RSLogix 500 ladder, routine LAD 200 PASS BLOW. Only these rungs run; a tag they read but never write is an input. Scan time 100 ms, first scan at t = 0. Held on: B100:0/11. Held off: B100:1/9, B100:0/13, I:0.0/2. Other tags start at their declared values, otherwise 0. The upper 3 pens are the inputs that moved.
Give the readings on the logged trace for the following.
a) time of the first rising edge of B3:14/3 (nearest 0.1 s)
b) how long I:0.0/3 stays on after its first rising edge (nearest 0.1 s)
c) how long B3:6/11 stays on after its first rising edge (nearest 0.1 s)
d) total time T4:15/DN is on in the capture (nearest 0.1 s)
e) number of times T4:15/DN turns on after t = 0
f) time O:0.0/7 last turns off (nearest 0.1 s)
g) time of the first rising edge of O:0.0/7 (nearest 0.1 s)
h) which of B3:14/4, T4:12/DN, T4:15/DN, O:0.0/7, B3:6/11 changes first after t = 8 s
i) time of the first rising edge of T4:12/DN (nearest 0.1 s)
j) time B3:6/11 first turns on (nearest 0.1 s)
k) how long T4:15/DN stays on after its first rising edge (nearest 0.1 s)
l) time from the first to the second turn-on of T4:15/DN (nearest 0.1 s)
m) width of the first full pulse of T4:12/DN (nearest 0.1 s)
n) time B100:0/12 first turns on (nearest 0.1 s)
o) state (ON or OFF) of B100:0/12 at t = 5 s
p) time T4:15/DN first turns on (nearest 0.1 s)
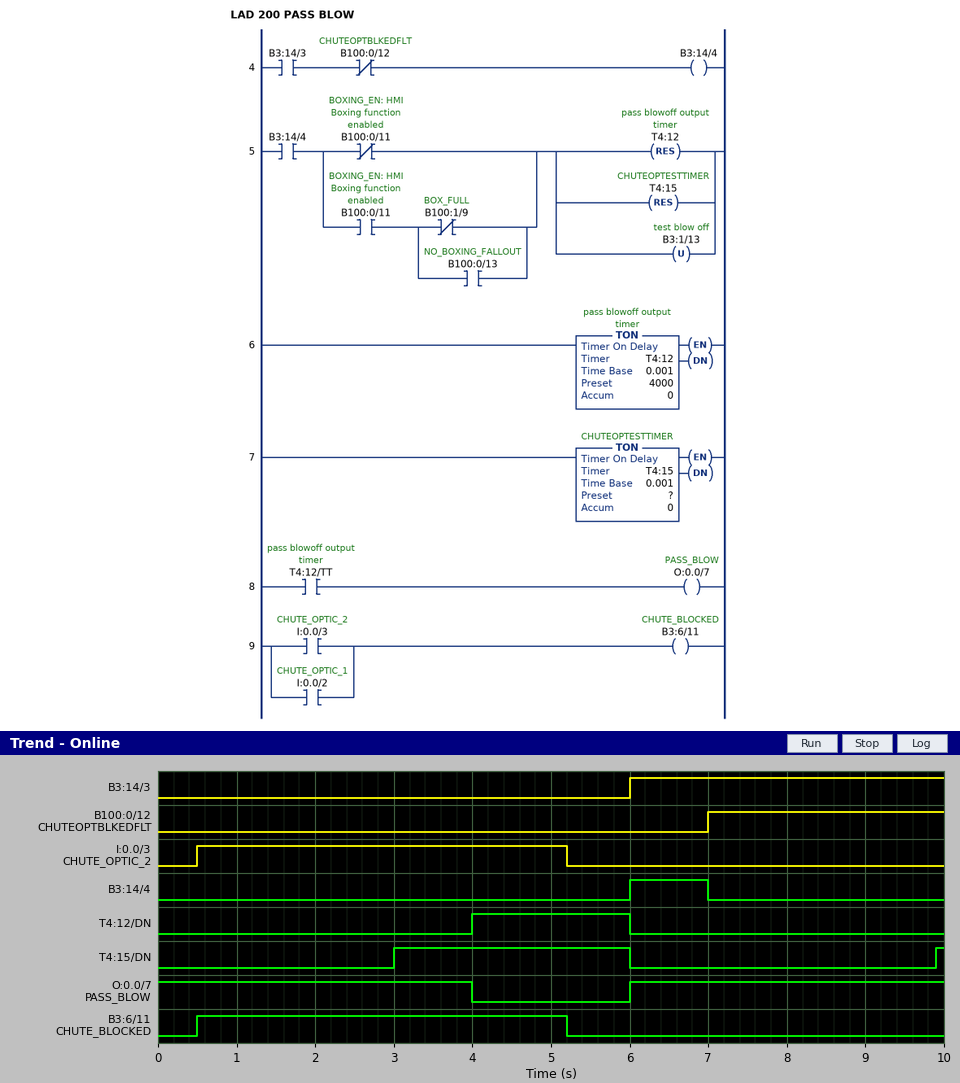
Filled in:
6.0 s
4.7 s
4.7 s
3.1 s
2
4.0 s
6.0 s
T4:15/DN
4.0 s
0.5 s
3.0 s
6.9 s
2.0 s
7.0 s
OFF
3.0 s
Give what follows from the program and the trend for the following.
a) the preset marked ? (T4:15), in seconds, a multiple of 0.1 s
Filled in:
3.0 s
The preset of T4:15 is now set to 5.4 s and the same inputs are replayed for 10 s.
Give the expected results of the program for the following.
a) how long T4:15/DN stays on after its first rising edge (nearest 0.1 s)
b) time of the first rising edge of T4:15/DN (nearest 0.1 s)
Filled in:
0.6 s
5.4 s
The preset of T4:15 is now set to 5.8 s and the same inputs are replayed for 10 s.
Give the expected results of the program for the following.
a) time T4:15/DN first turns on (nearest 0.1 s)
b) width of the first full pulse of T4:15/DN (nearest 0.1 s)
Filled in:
5.8 s
0.2 s
